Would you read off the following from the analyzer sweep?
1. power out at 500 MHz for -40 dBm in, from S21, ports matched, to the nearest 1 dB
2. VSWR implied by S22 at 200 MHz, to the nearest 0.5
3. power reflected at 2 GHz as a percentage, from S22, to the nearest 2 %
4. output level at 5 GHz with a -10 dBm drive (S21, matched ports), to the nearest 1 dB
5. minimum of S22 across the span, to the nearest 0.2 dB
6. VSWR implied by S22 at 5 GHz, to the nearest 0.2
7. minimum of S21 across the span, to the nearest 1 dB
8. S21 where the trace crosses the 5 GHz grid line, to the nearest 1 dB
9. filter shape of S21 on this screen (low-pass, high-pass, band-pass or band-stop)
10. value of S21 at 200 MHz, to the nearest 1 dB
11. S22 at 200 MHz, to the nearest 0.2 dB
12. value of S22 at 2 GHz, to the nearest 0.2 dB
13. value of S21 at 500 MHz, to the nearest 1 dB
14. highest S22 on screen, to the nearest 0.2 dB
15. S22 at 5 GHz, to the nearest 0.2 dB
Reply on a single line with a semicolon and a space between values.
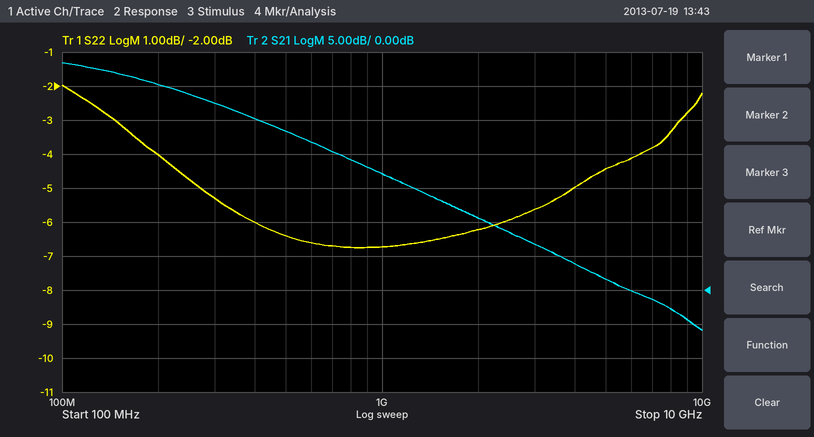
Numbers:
-17 dBm; 4.5; 24 %; -8 dBm; -6.8 dB; 4.0; -6 dB; 2 dB; low-pass; 30 dB; -4.0 dB; -6.2 dB; 23 dB; -2.0 dB; -4.4 dB
